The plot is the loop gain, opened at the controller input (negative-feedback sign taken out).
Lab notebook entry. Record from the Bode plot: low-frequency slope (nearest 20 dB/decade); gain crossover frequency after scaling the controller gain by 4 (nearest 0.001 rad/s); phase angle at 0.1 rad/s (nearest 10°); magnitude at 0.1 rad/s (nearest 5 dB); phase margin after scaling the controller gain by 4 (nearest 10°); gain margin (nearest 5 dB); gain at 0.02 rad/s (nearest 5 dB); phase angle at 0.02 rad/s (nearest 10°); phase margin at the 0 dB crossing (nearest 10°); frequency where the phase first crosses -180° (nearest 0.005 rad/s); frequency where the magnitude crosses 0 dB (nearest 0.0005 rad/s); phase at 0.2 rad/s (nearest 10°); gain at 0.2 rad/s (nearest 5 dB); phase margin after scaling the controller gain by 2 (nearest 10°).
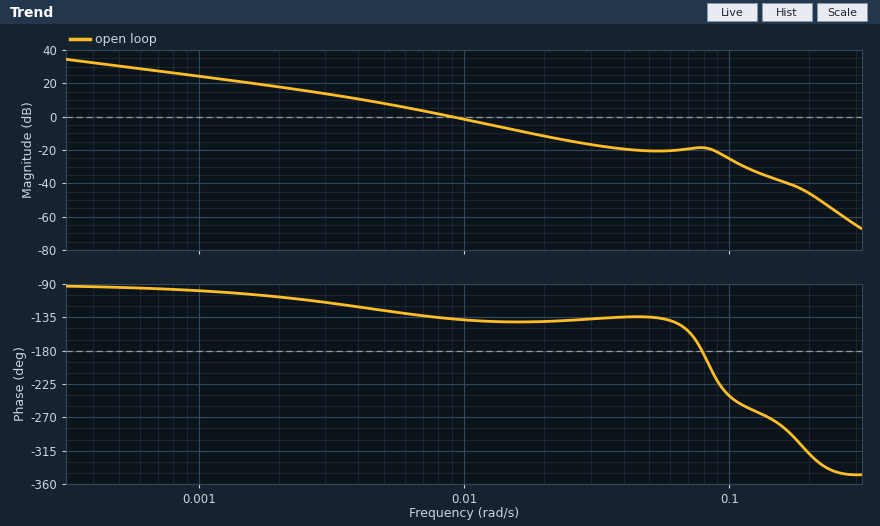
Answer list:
-20 dB/decade
0.021 rad/s
-240°
-25 dB
40°
20 dB
-10 dB
-140°
40°
0.080 rad/s
0.0090 rad/s
-320°
-45 dB
40°
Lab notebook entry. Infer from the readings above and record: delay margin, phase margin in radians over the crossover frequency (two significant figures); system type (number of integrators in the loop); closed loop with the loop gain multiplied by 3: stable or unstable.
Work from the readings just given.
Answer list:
78 s
1
stable
